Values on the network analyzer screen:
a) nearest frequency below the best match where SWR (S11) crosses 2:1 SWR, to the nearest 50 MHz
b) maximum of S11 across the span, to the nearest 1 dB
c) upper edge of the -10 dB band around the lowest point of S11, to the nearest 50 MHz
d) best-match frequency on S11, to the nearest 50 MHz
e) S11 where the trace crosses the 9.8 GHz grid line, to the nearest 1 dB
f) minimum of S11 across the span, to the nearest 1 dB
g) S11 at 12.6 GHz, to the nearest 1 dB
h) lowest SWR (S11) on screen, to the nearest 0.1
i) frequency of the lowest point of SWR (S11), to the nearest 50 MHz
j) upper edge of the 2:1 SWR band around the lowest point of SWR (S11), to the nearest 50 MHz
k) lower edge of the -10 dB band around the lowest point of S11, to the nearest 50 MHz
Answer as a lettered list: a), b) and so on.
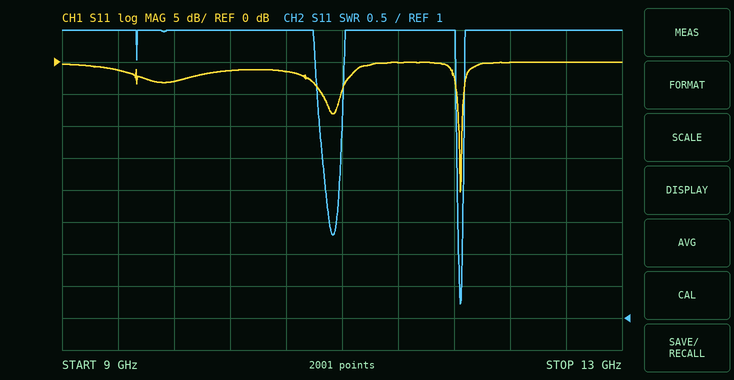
a) 11.85 GHz
b) 0 dB
c) 11.85 GHz
d) 11.85 GHz
e) -3 dB
f) -20 dB
g) 0 dB
h) 1.2
i) 11.85 GHz
j) 11.85 GHz
k) 11.85 GHz
